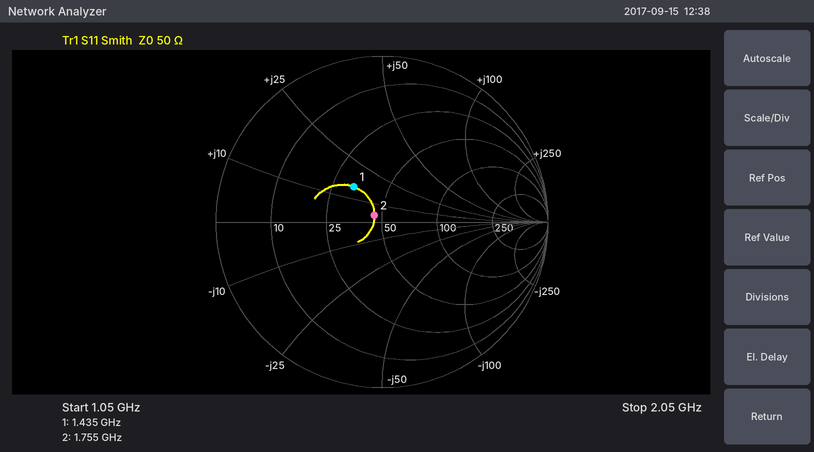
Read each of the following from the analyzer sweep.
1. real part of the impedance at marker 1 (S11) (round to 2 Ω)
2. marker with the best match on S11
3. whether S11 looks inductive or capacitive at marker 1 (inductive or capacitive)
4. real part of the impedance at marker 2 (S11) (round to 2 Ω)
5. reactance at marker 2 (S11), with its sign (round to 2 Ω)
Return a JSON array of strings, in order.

["32 Ω", "marker 2", "inductive", "46 Ω", "+4 Ω"]
